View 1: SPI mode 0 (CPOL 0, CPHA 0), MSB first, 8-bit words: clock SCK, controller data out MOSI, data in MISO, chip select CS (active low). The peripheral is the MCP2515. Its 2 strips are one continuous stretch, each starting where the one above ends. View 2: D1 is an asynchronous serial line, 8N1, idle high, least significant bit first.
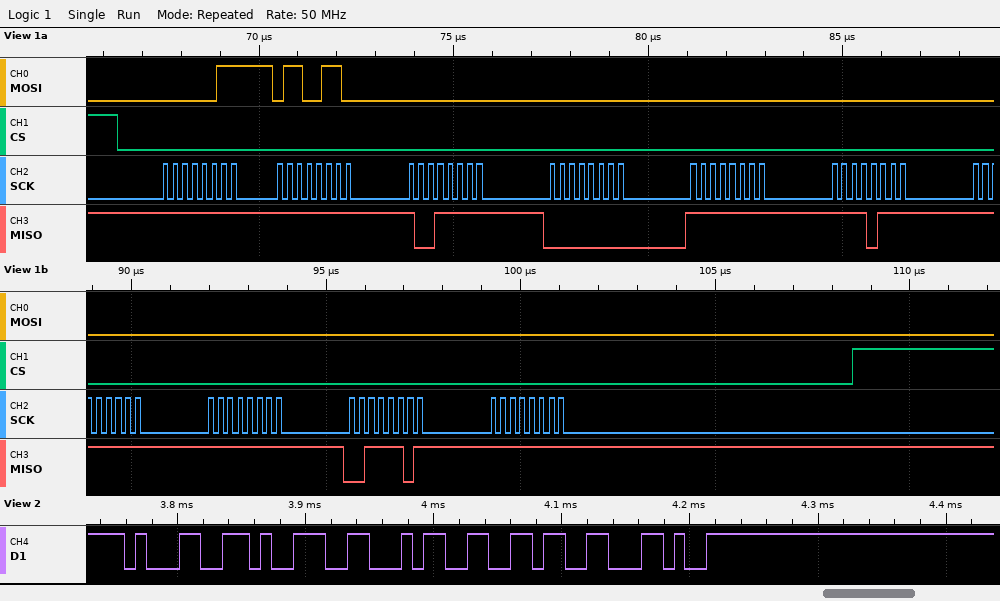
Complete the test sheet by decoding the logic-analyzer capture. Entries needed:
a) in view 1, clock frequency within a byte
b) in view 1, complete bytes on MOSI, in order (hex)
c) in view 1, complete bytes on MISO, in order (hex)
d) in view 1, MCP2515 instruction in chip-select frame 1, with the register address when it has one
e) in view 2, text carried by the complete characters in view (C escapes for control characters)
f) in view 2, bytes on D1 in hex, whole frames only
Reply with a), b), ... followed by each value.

a) 4 MHz
b) 03 66 00 00 00 00 00 00 00 00
c) FF FF 9F 00 FF F7 FF FF 3D FF
d) READ 0x66
e) "1946,"
f) 0x31 0x39 0x34 0x36 0x2C
